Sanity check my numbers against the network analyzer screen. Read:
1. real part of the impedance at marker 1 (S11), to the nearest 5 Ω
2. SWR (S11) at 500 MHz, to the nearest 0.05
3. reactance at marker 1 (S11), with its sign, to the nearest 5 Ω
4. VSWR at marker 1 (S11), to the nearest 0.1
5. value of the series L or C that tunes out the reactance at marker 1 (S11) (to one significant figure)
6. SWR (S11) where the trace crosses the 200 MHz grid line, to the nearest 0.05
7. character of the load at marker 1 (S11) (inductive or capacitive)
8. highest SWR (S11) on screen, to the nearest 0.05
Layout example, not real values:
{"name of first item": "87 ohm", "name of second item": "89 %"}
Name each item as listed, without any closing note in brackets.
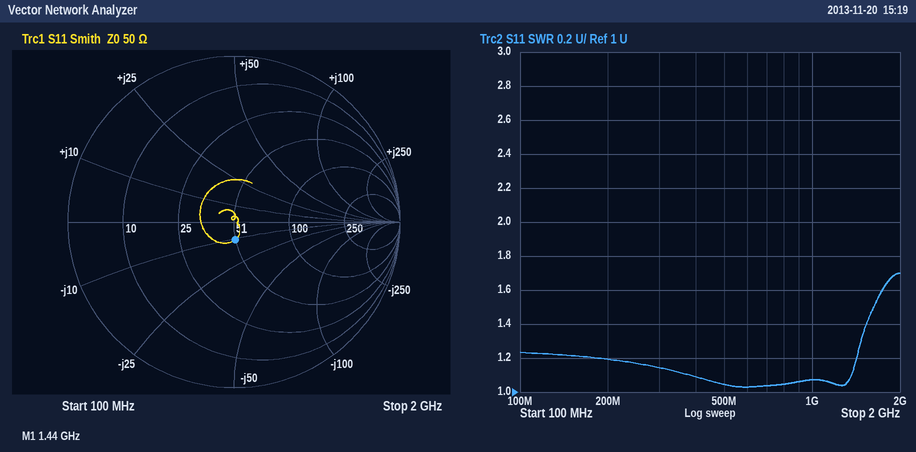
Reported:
{"real part of the impedance at marker 1 (S11), to the nearest 5 Ω": "50 Ω", "SWR (S11) at 500 MHz, to the nearest 0.05": "1.05", "reactance at marker 1 (S11), with its sign, to the nearest 5 Ω": "-10 Ω", "VSWR at marker 1 (S11), to the nearest 0.1": "1.2", "value of the series L or C that tunes out the reactance at marker 1 (S11)": "1 nH", "SWR (S11) where the trace crosses the 200 MHz grid line, to the nearest 0.05": "1.20", "character of the load at marker 1 (S11)": "capacitive", "highest SWR (S11) on screen, to the nearest 0.05": "1.70"}
